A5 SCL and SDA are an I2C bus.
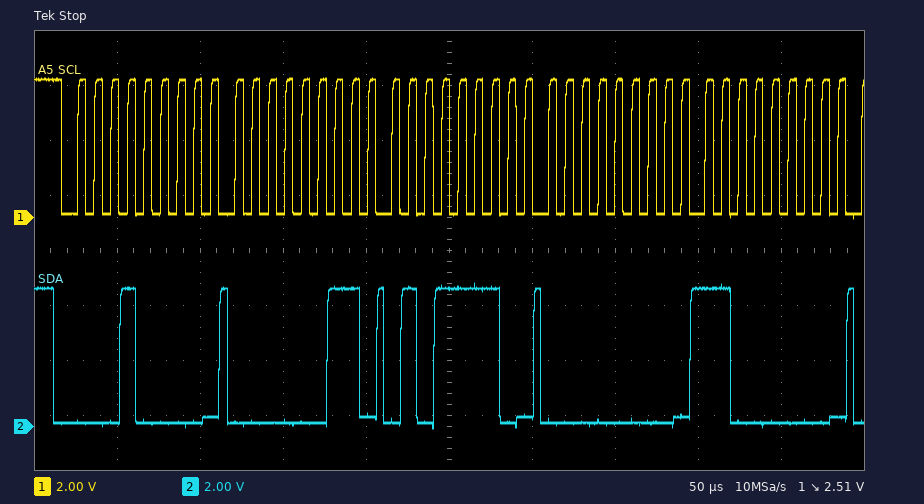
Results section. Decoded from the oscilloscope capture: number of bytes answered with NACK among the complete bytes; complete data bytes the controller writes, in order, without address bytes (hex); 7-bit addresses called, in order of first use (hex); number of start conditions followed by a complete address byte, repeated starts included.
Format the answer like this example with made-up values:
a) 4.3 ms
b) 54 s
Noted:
a) 0
b) 03 5E 00 C0
c) 0x08
d) 1
